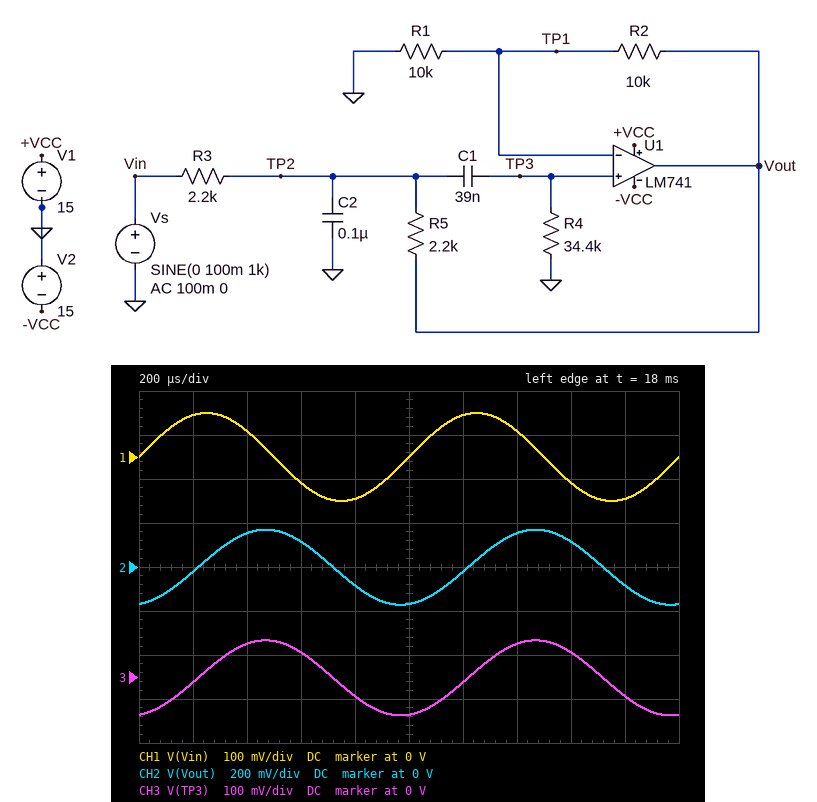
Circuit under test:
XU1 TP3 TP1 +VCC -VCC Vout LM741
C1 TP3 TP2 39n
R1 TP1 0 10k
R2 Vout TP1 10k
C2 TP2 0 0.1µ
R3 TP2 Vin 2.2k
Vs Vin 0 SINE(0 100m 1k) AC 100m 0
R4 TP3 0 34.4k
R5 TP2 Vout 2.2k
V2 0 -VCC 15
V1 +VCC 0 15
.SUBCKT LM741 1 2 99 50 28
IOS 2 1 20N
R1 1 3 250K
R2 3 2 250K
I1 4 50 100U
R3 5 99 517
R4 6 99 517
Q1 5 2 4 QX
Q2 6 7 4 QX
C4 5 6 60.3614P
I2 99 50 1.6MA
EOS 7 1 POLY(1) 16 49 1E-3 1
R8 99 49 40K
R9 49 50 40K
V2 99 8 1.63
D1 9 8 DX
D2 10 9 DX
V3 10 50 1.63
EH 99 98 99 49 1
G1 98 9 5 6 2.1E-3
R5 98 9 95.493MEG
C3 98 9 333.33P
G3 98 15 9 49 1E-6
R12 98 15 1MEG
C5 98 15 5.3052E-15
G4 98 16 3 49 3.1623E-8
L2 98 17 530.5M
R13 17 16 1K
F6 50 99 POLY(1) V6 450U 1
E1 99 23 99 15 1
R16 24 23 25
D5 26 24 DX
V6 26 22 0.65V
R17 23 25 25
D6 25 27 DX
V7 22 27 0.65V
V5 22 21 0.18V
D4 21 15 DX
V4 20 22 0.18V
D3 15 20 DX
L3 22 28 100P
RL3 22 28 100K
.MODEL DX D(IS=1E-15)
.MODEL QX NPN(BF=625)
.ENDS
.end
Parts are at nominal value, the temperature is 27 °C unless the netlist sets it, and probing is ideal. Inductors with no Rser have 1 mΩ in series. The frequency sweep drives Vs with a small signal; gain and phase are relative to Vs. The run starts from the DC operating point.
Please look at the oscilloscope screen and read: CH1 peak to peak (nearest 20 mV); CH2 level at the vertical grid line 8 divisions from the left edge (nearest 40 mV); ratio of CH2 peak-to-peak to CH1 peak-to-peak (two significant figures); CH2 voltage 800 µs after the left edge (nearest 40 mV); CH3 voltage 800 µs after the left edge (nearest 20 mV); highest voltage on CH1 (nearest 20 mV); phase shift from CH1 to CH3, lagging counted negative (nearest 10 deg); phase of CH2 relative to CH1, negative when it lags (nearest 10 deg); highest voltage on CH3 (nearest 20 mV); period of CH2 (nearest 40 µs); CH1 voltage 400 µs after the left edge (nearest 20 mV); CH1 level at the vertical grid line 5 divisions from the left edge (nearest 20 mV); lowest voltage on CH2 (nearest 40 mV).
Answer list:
200 mV
120 mV
1.7
-80 mV
-40 mV
100 mV
-80 deg
-80 deg
80 mV
1.00 ms
60 mV
0 V
-160 mV
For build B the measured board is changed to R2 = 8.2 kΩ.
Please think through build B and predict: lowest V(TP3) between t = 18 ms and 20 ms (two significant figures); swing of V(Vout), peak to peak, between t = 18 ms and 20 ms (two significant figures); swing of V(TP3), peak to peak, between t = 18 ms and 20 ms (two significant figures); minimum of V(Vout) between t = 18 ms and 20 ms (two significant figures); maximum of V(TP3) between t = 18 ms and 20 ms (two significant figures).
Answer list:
-84 mV
300 mV
160 mV
-150 mV
80 mV
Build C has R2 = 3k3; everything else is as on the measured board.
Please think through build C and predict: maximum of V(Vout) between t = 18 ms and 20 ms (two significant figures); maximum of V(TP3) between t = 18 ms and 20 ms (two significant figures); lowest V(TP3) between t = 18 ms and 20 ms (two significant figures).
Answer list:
90 mV
67 mV
-71 mV
